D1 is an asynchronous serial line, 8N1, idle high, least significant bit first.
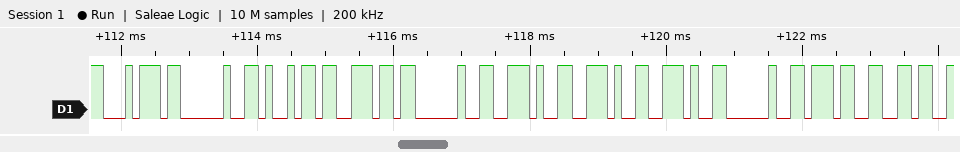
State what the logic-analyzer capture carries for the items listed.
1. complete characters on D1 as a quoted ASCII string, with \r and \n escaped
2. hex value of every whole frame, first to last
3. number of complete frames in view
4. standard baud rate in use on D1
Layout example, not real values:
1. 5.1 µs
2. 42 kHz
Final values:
1. "t in ... 76"
2. 0x74 0x20 0x69 0x6E 0x20 0x2E 0x2E 0x2E 0x20 0x37 0x36
3. 11
4. 9600 baud
